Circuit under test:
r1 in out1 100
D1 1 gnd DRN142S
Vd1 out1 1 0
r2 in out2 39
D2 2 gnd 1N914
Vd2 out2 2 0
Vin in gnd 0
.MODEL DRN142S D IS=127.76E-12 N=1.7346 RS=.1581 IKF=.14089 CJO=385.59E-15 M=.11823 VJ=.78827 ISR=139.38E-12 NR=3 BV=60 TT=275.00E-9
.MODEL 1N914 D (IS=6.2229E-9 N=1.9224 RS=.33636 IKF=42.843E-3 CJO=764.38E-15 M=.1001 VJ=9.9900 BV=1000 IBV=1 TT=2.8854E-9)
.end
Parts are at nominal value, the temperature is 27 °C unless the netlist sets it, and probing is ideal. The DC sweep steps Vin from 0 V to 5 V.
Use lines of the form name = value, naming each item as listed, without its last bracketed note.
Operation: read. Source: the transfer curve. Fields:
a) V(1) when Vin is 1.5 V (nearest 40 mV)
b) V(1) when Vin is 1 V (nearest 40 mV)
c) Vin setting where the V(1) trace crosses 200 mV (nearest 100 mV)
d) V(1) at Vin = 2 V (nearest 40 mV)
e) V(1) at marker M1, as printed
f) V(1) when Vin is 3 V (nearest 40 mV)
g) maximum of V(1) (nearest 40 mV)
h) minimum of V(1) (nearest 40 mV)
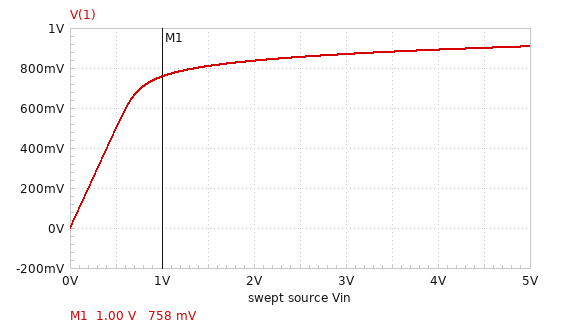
V(1) when Vin is 1.5 V = 800 mV
V(1) when Vin is 1 V = 760 mV
Vin setting where the V(1) trace crosses 200 mV = 200 mV
V(1) at Vin = 2 V = 840 mV
V(1) at marker M1, as printed = 758 mV
V(1) when Vin is 3 V = 880 mV
maximum of V(1) = 920 mV
minimum of V(1) = 0 V
